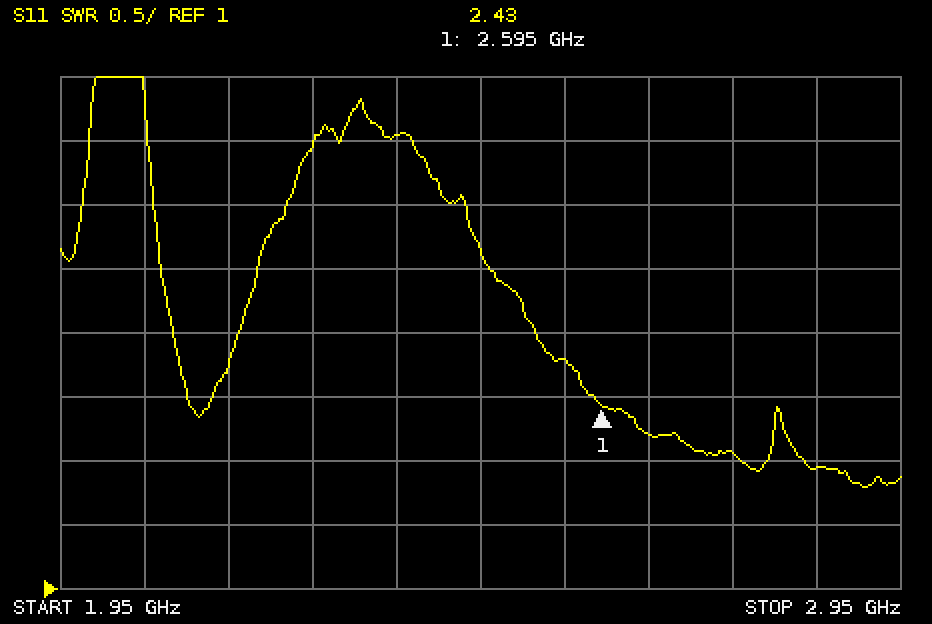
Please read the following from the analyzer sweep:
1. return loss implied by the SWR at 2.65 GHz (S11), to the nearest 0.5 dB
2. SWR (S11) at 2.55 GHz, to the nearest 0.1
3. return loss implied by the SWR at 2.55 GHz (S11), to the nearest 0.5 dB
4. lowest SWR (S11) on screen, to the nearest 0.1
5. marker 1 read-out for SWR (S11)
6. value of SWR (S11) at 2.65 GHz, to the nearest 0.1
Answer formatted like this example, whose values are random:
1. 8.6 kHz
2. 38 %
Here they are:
1. 8.5 dB
2. 2.8
3. 6.5 dB
4. 1.8
5. 2.43
6. 2.2
